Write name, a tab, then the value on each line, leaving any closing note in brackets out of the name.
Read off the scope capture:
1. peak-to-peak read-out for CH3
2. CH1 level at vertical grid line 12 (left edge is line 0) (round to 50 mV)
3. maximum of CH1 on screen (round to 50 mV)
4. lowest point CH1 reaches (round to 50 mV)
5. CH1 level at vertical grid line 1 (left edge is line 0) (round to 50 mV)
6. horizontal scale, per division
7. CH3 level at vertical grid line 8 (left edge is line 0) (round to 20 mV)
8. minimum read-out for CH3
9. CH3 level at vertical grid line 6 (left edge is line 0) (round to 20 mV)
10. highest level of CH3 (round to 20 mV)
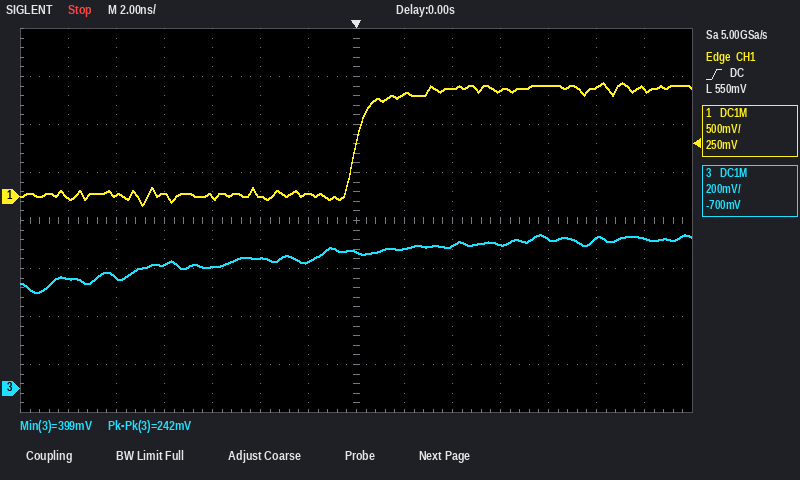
peak-to-peak read-out for CH3	242 mV
CH1 level at vertical grid line 12 (left edge is line 0)	1.15 V
maximum of CH1 on screen	1.20 V
lowest point CH1 reaches	-100 mV
CH1 level at vertical grid line 1 (left edge is line 0)	0 mV
horizontal scale, per division	2 ns
CH3 level at vertical grid line 8 (left edge is line 0)	580 mV
minimum read-out for CH3	399 mV
CH3 level at vertical grid line 6 (left edge is line 0)	520 mV
highest level of CH3	640 mV
